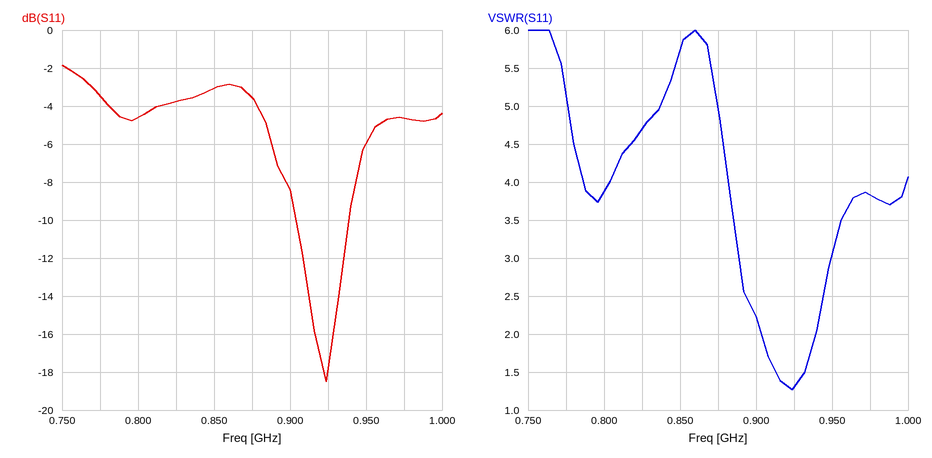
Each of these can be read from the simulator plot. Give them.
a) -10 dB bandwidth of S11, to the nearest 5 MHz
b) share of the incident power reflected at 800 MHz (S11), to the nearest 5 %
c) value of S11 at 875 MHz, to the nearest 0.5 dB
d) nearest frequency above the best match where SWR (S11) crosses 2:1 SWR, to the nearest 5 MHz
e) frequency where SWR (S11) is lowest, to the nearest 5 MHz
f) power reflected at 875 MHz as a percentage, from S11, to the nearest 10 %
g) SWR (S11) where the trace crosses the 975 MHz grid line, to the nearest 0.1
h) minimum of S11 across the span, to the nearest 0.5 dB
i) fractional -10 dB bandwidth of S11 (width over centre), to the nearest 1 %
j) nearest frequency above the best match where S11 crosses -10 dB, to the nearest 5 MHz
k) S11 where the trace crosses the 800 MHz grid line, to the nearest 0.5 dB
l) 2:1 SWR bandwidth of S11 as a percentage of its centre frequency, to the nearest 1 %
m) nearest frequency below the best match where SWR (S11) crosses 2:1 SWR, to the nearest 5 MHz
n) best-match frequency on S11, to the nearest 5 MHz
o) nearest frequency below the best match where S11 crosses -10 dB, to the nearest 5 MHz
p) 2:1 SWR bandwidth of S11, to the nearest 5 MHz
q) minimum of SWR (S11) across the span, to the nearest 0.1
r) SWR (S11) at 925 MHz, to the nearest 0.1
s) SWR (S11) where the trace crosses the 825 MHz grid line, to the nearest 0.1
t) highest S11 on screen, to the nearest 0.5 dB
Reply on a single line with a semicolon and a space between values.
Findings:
35 MHz; 35 %; -3.5 dB; 940 MHz; 925 MHz; 40 %; 3.8; -18.5 dB; 4 %; 940 MHz; -4.5 dB; 4 %; 905 MHz; 925 MHz; 905 MHz; 35 MHz; 1.3; 1.3; 4.7; -2.0 dB
